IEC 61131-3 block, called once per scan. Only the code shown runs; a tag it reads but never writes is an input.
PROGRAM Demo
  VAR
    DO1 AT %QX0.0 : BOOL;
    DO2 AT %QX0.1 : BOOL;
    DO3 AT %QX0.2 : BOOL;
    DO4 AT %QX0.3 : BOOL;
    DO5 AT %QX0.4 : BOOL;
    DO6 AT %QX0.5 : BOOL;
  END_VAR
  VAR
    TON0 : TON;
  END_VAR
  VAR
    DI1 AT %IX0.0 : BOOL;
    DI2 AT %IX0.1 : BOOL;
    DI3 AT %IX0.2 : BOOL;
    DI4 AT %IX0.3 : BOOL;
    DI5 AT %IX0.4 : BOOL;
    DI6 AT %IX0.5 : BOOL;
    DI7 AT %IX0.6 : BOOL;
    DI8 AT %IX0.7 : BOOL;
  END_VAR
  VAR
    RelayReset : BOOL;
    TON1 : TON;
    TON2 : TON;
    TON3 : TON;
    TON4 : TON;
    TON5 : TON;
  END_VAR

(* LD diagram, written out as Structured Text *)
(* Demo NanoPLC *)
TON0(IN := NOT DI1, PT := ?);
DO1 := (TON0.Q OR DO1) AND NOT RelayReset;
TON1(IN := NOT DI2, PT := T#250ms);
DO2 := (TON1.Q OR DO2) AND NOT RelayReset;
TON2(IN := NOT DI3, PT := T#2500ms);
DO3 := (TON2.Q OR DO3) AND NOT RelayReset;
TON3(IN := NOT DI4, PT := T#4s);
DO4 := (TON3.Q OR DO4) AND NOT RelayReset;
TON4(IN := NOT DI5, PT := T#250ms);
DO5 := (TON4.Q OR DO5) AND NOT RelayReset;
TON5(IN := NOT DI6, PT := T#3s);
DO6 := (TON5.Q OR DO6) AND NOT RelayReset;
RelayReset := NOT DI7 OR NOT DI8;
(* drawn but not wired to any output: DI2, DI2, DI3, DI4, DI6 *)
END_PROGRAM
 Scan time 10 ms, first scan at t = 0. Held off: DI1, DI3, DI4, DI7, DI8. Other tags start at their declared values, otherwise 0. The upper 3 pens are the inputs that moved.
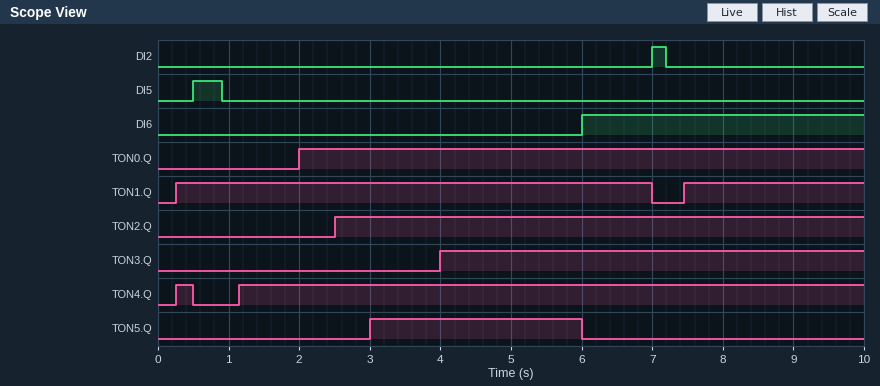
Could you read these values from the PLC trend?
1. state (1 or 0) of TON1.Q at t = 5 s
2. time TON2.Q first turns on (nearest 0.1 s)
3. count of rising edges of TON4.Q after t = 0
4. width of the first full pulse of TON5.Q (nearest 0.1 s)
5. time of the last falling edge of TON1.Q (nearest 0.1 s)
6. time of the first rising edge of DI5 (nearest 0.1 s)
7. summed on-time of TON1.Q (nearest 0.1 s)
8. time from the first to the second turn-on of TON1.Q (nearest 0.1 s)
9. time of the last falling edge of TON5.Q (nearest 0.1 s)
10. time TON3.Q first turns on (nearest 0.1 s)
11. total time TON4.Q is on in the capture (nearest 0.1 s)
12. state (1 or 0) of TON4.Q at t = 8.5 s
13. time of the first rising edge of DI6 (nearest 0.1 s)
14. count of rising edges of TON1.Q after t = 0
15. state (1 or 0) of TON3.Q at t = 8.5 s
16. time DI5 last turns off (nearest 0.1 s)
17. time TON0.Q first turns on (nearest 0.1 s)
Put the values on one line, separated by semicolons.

1; 2.5 s; 2; 3.0 s; 7.0 s; 0.5 s; 9.3 s; 7.2 s; 6.0 s; 4.0 s; 9.1 s; 1; 6.0 s; 2; 1; 0.9 s; 2.0 s
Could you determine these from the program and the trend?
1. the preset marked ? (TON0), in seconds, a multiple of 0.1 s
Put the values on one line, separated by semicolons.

2.0 s
